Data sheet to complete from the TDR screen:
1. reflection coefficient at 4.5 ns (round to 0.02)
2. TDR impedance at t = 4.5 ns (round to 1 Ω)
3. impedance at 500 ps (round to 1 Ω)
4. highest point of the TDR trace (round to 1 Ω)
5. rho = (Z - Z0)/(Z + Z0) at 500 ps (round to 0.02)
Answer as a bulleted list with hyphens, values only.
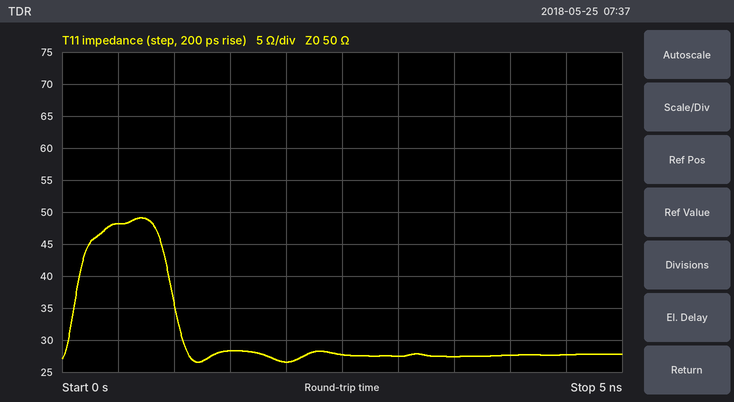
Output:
- -0.28
- 28 Ω
- 48 Ω
- 49 Ω
- -0.02
